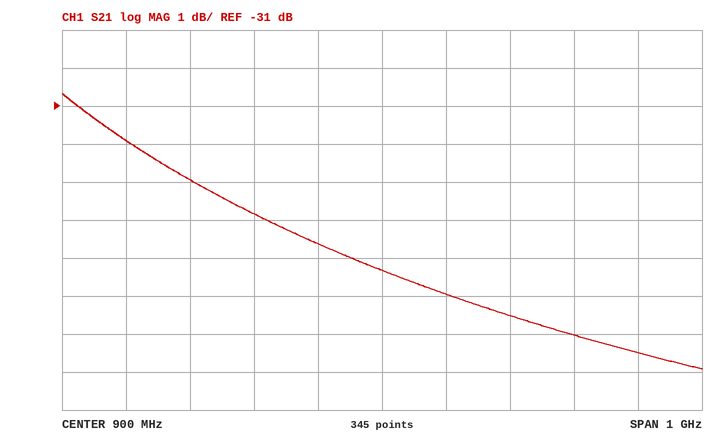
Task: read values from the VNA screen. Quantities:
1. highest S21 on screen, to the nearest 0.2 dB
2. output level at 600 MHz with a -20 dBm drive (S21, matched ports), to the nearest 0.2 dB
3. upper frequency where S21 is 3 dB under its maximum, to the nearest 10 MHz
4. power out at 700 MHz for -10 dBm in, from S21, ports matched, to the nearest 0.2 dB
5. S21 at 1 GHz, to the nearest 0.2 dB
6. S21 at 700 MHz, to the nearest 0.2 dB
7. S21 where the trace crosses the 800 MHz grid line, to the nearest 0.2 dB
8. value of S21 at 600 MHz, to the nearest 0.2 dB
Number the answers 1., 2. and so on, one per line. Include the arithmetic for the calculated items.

1. -30.6 dB
2. -20 dBm + (-33.0 dB) = -53.0 dBm
3. 680 MHz
4. -10 dBm + (-33.8 dB) = -43.8 dBm
5. -36.0 dB
6. -33.8 dB
7. -34.6 dB
8. -33.0 dB
